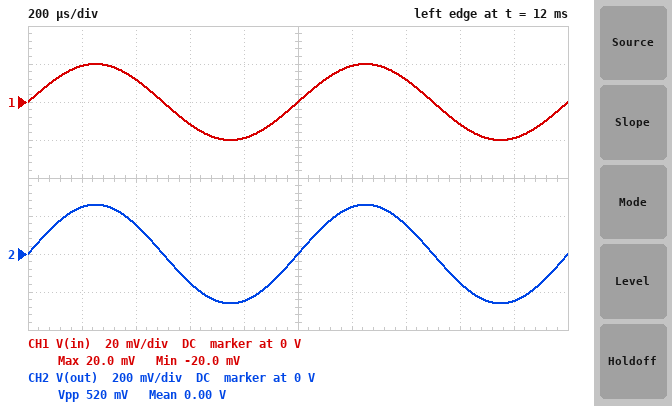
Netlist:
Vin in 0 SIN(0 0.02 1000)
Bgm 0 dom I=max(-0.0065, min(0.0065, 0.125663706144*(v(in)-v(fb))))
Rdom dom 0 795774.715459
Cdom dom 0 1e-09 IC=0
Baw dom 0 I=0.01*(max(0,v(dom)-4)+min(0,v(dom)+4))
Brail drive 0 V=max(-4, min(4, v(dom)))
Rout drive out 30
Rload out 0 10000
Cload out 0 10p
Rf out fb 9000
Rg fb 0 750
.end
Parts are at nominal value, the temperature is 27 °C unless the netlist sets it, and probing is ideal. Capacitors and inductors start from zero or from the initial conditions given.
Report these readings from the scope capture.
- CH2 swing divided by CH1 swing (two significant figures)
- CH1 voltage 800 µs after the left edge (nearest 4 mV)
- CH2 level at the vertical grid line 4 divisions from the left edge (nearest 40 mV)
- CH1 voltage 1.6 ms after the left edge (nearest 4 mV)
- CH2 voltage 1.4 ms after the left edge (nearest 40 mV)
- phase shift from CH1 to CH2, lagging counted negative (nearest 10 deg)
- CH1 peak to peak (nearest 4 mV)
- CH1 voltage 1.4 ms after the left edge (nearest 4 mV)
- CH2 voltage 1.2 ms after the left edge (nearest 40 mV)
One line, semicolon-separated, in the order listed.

13; -20 mV; -240 mV; -12 mV; 160 mV; 0 deg; 40 mV; 12 mV; 240 mV
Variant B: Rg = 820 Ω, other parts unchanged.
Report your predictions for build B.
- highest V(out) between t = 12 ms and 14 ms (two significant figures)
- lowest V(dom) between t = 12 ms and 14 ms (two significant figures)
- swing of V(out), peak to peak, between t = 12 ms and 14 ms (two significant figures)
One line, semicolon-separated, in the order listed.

240 mV; -240 mV; 480 mV
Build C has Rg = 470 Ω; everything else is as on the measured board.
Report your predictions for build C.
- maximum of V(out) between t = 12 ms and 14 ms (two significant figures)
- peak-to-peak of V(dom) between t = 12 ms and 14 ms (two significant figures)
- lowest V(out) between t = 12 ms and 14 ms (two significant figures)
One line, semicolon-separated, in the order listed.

400 mV; 810 mV; -400 mV
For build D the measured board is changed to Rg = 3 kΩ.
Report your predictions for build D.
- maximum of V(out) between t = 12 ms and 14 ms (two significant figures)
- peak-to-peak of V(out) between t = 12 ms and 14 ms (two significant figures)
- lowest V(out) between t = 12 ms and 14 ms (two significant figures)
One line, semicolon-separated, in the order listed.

80 mV; 160 mV; -80 mV
